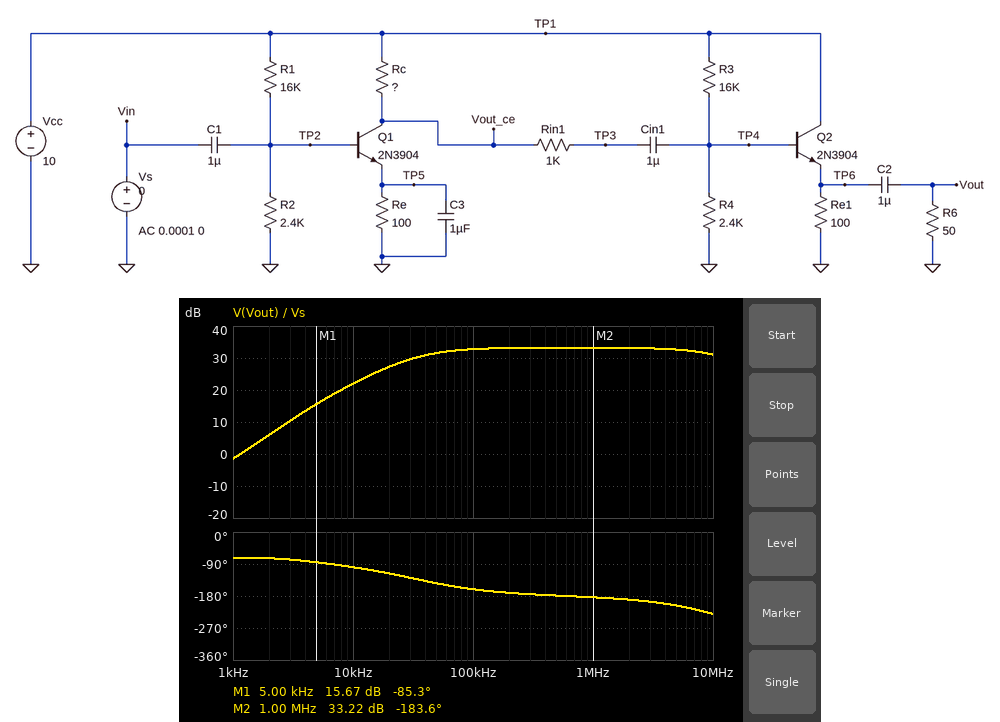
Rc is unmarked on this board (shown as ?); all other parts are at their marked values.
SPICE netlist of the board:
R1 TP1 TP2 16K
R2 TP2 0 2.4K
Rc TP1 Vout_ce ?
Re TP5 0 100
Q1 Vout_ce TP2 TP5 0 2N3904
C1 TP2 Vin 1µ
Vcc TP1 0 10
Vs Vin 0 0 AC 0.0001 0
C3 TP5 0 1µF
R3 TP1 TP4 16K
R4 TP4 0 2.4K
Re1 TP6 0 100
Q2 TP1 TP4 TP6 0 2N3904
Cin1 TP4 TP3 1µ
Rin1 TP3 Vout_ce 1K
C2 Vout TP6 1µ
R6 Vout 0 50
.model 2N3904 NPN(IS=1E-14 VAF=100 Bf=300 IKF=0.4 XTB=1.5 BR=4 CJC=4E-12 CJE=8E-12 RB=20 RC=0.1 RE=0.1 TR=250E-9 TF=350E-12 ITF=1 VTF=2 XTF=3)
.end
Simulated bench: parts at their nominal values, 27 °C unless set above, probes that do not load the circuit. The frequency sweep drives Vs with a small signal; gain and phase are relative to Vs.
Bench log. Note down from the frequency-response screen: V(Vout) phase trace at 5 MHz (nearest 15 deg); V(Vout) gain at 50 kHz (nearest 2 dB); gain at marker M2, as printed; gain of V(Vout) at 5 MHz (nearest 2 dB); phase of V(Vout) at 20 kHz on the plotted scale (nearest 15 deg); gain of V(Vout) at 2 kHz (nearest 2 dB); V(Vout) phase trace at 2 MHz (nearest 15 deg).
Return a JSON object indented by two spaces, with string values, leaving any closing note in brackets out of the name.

{
  "V(Vout) phase trace at 5 MHz": "-210 deg",
  "V(Vout) gain at 50 kHz": "32 dB",
  "gain at marker M2, as printed": "33.22 dB",
  "gain of V(Vout) at 5 MHz": "32 dB",
  "phase of V(Vout) at 20 kHz on the plotted scale": "-120 deg",
  "gain of V(Vout) at 2 kHz": "6 dB",
  "V(Vout) phase trace at 2 MHz": "-195 deg"
}
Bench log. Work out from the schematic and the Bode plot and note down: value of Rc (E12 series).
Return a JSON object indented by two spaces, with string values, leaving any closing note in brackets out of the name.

{
  "value of Rc": "470 Ω"
}
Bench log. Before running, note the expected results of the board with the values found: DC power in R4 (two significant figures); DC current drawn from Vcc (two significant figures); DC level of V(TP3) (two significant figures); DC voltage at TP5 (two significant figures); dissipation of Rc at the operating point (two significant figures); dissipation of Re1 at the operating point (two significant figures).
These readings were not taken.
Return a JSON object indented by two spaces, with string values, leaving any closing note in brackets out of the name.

{
  "DC power in R4": "670 µW",
  "DC current drawn from Vcc": "12 mA",
  "DC level of V(TP3)": "7.3 V",
  "DC voltage at TP5": "570 mV",
  "dissipation of Rc at the operating point": "15 mW",
  "dissipation of Re1 at the operating point": "3.2 mW"
}
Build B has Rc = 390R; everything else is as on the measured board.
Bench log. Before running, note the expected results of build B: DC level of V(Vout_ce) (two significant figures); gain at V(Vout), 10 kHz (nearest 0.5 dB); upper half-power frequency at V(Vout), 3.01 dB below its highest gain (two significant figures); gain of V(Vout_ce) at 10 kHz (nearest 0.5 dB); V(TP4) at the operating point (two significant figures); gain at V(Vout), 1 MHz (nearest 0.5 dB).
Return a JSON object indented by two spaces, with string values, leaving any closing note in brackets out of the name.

{
  "DC level of V(Vout_ce)": "7.8 V",
  "gain at V(Vout), 10 kHz": "20.5 dB",
  "upper half-power frequency at V(Vout), 3.01 dB below its highest gain": "13 MHz",
  "gain of V(Vout_ce) at 10 kHz": "26.0 dB",
  "V(TP4) at the operating point": "1.3 V",
  "gain at V(Vout), 1 MHz": "32.0 dB"
}
